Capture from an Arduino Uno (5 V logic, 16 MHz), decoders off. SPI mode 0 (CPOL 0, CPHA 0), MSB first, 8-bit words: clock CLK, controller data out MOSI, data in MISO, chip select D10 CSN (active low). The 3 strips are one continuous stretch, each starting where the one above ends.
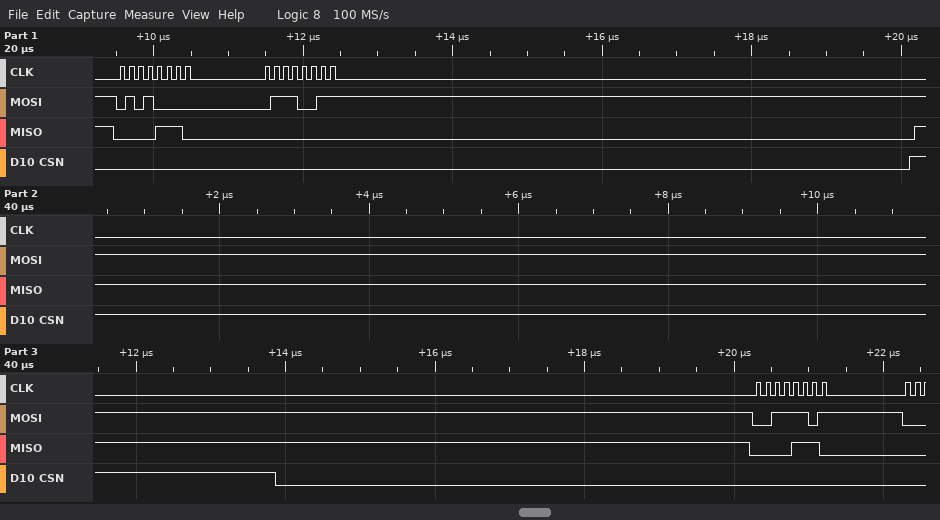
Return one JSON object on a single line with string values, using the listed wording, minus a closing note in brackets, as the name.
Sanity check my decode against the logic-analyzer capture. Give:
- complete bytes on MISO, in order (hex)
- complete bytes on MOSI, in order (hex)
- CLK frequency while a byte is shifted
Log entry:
{"complete bytes on MISO, in order": "0E 00 0E", "complete bytes on MOSI, in order": "50 73 3D", "CLK frequency while a byte is shifted": "8 MHz"}
